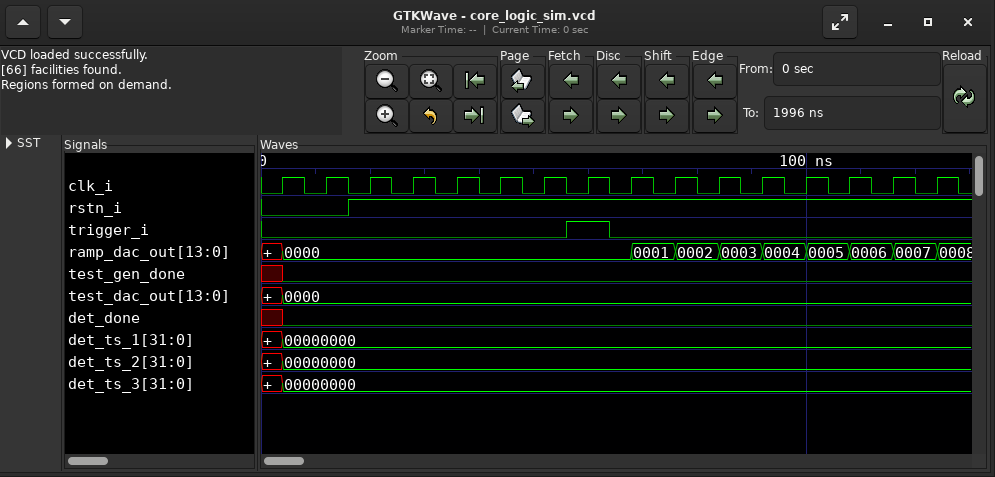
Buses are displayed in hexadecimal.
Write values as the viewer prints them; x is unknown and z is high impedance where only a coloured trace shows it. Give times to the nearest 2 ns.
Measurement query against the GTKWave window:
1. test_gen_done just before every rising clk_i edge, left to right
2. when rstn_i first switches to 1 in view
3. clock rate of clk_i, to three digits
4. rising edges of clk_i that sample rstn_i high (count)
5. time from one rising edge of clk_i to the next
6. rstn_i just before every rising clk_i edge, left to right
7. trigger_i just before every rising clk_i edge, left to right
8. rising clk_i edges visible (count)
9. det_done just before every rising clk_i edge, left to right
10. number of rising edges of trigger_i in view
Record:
x 0 0 0 0 0 0 0 0 0 0 0 0 0 0 0
16 ns
125 MHz
14
8 ns
0 0 1 1 1 1 1 1 1 1 1 1 1 1 1 1
0 0 0 0 0 0 0 1 0 0 0 0 0 0 0 0
16
x 0 0 0 0 0 0 0 0 0 0 0 0 0 0 0
1
